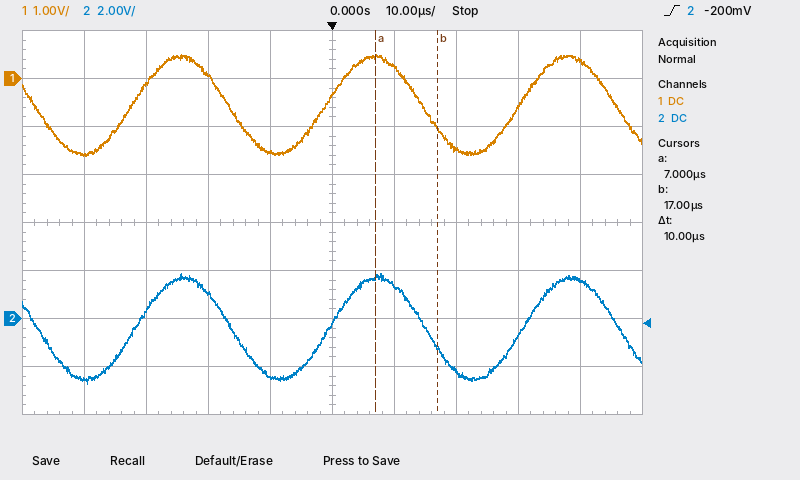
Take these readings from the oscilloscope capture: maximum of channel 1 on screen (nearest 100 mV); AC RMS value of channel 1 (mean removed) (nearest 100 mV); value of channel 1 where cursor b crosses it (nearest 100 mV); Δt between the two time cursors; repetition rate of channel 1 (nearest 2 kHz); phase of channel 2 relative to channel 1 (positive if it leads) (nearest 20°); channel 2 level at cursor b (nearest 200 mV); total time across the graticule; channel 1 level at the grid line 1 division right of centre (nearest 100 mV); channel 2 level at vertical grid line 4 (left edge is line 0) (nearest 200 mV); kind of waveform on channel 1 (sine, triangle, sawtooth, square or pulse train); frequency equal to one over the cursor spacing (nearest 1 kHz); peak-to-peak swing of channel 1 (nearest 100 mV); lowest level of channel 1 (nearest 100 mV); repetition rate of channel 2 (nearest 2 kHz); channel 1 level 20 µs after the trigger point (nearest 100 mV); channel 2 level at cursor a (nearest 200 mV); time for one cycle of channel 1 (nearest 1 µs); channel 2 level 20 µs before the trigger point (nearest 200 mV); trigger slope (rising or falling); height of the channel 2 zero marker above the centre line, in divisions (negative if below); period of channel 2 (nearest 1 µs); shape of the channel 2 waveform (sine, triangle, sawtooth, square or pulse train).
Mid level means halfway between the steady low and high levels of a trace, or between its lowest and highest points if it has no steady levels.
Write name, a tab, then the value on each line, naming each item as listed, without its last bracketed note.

maximum of channel 1 on screen	500 mV
AC RMS value of channel 1 (mean removed)	700 mV
value of channel 1 where cursor b crosses it	-1.0 V
Δt between the two time cursors	10 µs
repetition rate of channel 1	32 kHz
phase of channel 2 relative to channel 1 (positive if it leads)	0°
channel 2 level at cursor b	-1.2 V
total time across the graticule	100 µs
channel 1 level at the grid line 1 division right of centre	200 mV
channel 2 level at vertical grid line 4 (left edge is line 0)	-2.4 V
kind of waveform on channel 1	sine
frequency equal to one over the cursor spacing	100 kHz
peak-to-peak swing of channel 1	2.1 V
lowest level of channel 1	-1.6 V
repetition rate of channel 2	32 kHz
channel 1 level 20 µs after the trigger point	-1.5 V
channel 2 level at cursor a	1.8 V
time for one cycle of channel 1	31 µs
channel 2 level 20 µs before the trigger point	1.0 V
trigger slope	rising
height of the channel 2 zero marker above the centre line, in divisions	-2.0 div
period of channel 2	31 µs
shape of the channel 2 waveform	sine
